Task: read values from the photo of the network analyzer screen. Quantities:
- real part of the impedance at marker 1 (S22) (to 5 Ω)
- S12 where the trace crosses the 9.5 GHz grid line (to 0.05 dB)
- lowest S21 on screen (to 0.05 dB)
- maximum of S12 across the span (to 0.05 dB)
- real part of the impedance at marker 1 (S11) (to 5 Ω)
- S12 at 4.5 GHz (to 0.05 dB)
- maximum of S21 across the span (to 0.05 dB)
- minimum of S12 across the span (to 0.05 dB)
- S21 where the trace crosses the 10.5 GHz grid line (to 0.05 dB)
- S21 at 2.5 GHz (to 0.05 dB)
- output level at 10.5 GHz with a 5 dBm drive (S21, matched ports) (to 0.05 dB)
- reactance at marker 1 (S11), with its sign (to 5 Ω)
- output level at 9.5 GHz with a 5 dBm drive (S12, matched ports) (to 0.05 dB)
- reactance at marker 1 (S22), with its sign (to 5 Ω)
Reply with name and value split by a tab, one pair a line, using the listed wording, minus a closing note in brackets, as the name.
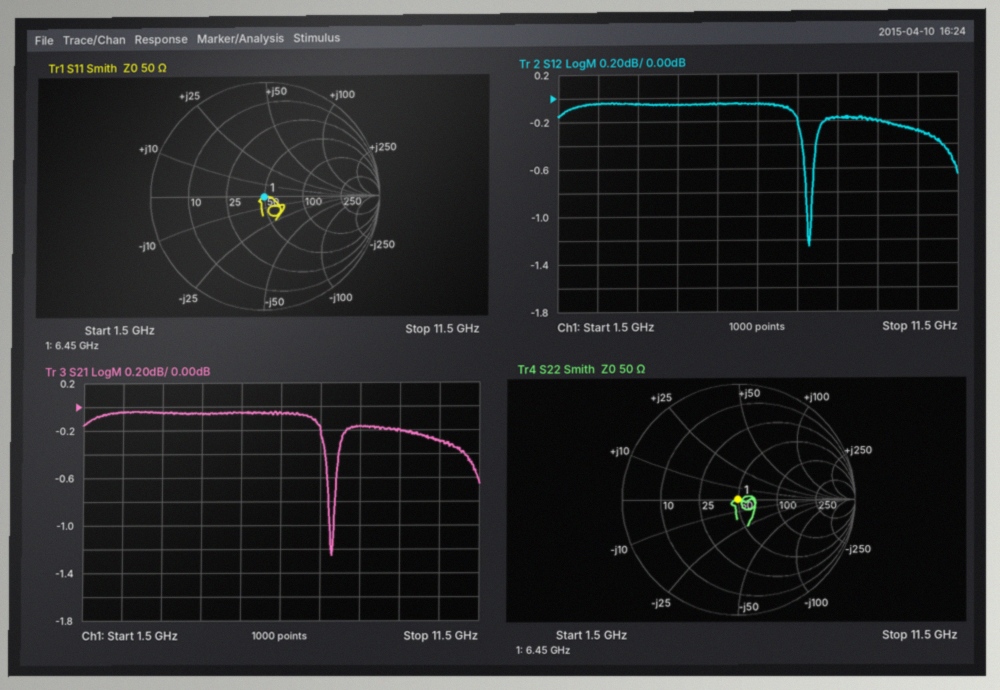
real part of the impedance at marker 1 (S22)	50 Ω
S12 where the trace crosses the 9.5 GHz grid line	-0.20 dB
lowest S21 on screen	-1.25 dB
maximum of S12 across the span	-0.05 dB
real part of the impedance at marker 1 (S11)	50 Ω
S12 at 4.5 GHz	-0.05 dB
maximum of S21 across the span	-0.05 dB
minimum of S12 across the span	-1.25 dB
S21 where the trace crosses the 10.5 GHz grid line	-0.30 dB
S21 at 2.5 GHz	-0.05 dB
output level at 10.5 GHz with a 5 dBm drive (S21, matched ports)	4.70 dBm
reactance at marker 1 (S11), with its sign	0 Ω
output level at 9.5 GHz with a 5 dBm drive (S12, matched ports)	4.80 dBm
reactance at marker 1 (S22), with its sign	0 Ω
